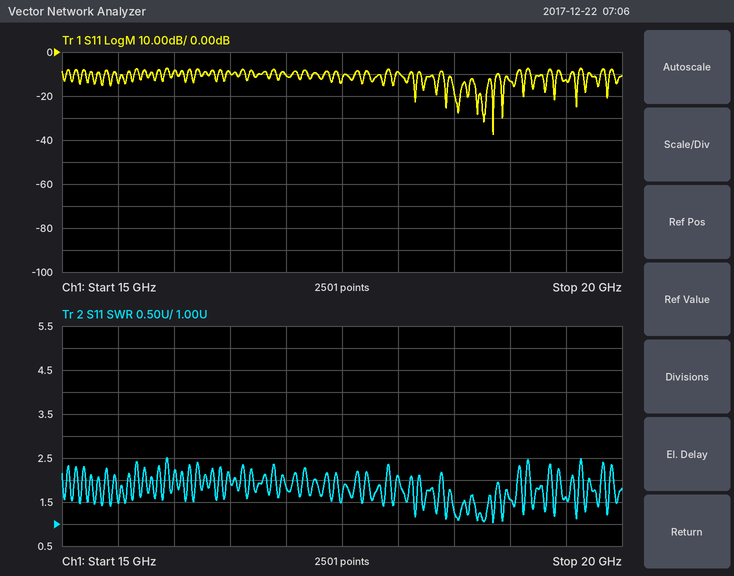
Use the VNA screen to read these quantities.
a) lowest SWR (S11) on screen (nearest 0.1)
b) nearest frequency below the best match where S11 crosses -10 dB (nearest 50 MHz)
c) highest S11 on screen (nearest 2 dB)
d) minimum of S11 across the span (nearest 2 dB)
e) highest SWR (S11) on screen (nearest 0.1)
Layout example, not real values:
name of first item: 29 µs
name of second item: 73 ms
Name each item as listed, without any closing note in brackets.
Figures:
lowest SWR (S11) on screen: 1.0
nearest frequency below the best match where S11 crosses -10 dB: 18.40 GHz
highest S11 on screen: -8 dB
minimum of S11 across the span: -38 dB
highest SWR (S11) on screen: 2.5
